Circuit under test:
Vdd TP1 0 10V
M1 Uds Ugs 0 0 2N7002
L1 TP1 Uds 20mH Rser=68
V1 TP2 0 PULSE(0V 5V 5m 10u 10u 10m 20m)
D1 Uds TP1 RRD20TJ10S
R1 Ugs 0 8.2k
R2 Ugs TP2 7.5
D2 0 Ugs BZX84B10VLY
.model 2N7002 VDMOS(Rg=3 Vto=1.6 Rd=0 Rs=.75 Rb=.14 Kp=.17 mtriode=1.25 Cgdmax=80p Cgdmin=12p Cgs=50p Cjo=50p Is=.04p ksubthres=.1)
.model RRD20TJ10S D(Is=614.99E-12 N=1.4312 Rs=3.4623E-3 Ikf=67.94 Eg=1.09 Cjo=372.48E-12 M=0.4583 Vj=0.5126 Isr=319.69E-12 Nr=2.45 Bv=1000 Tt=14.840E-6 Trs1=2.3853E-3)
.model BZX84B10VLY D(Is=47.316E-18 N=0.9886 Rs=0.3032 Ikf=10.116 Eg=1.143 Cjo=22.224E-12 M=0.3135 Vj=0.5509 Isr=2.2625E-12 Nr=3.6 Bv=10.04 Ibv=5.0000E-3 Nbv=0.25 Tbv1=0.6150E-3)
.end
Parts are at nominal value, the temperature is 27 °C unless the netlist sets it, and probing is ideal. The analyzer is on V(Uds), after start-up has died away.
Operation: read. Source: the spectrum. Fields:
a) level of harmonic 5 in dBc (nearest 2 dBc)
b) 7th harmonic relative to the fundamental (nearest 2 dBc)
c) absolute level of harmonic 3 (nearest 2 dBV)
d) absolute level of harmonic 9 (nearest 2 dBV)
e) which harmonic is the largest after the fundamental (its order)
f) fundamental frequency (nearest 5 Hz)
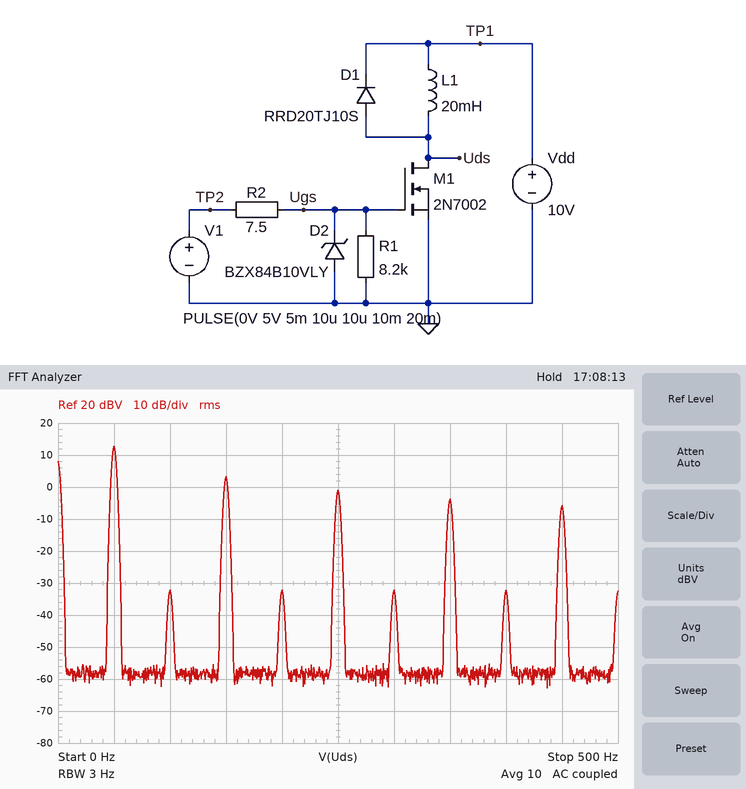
-14 dBc
-16 dBc
4 dBV
-6 dBV
3
50 Hz
